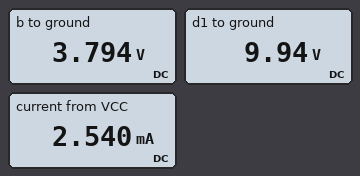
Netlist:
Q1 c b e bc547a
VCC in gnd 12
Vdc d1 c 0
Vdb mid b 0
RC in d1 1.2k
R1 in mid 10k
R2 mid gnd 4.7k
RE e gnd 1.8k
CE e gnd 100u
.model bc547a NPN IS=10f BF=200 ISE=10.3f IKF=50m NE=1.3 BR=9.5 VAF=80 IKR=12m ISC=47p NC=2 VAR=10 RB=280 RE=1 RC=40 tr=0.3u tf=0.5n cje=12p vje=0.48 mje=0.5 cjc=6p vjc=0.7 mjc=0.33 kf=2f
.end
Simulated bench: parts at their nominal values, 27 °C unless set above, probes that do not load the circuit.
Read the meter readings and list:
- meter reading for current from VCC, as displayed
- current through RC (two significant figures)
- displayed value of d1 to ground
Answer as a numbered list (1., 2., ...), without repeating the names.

1. 2.540 mA
2. 1.7 mA
3. 9.94 V
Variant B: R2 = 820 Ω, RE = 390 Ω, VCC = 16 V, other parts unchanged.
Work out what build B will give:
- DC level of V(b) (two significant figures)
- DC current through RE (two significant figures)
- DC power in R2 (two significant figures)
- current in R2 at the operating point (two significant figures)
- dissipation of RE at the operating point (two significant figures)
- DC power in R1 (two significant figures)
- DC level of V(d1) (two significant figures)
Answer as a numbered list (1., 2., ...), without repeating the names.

1. 1.2 V
2. 1.4 mA
3. 1.8 mW
4. 1.5 mA
5. 750 µW
6. 22 mW
7. 14 V
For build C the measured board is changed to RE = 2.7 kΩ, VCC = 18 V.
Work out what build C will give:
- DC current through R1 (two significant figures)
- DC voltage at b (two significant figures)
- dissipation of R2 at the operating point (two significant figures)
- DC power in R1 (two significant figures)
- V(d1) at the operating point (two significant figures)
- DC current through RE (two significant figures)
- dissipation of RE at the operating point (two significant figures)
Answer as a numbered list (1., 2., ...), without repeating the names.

1. 1.2 mA
2. 5.7 V
3. 6.9 mW
4. 15 mW
5. 16 V
6. 1.9 mA
7. 9.4 mW
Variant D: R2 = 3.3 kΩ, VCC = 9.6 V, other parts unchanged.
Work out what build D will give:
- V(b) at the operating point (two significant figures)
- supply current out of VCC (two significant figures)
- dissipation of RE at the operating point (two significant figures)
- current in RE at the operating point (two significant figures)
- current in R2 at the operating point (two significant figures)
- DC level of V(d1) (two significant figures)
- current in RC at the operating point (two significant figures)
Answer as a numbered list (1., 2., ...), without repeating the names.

1. 2.4 V
2. 1.7 mA
3. 1.6 mW
4. 950 µA
5. 720 µA
6. 8.5 V
7. 940 µA
